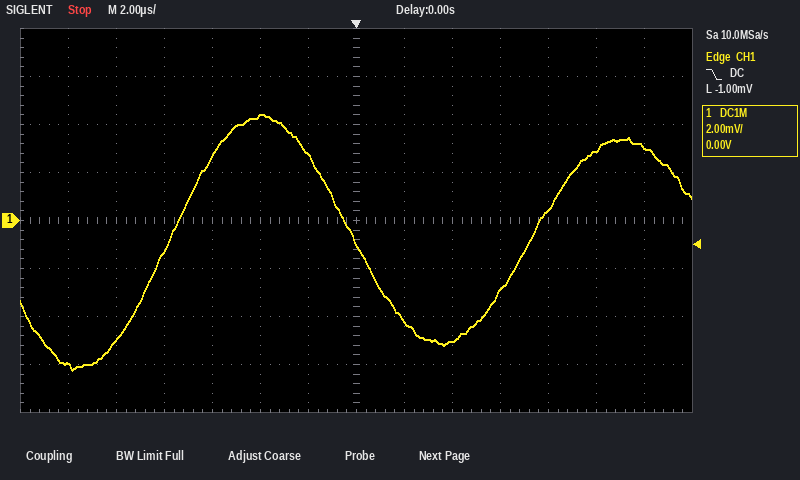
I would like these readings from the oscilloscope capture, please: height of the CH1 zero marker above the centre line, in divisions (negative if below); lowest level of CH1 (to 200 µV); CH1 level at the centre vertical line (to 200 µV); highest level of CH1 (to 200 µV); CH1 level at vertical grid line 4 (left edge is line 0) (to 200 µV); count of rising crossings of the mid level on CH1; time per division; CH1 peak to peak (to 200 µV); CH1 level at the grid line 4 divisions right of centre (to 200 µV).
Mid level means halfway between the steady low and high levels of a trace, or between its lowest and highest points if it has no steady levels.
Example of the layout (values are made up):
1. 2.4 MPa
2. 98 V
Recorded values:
1. 0.0 div
2. -6.2 mV
3. -1.0 mV
4. 4.4 mV
5. 2.6 mV
6. 2
7. 2 µs
8. 10.6 mV
9. 400 µV
